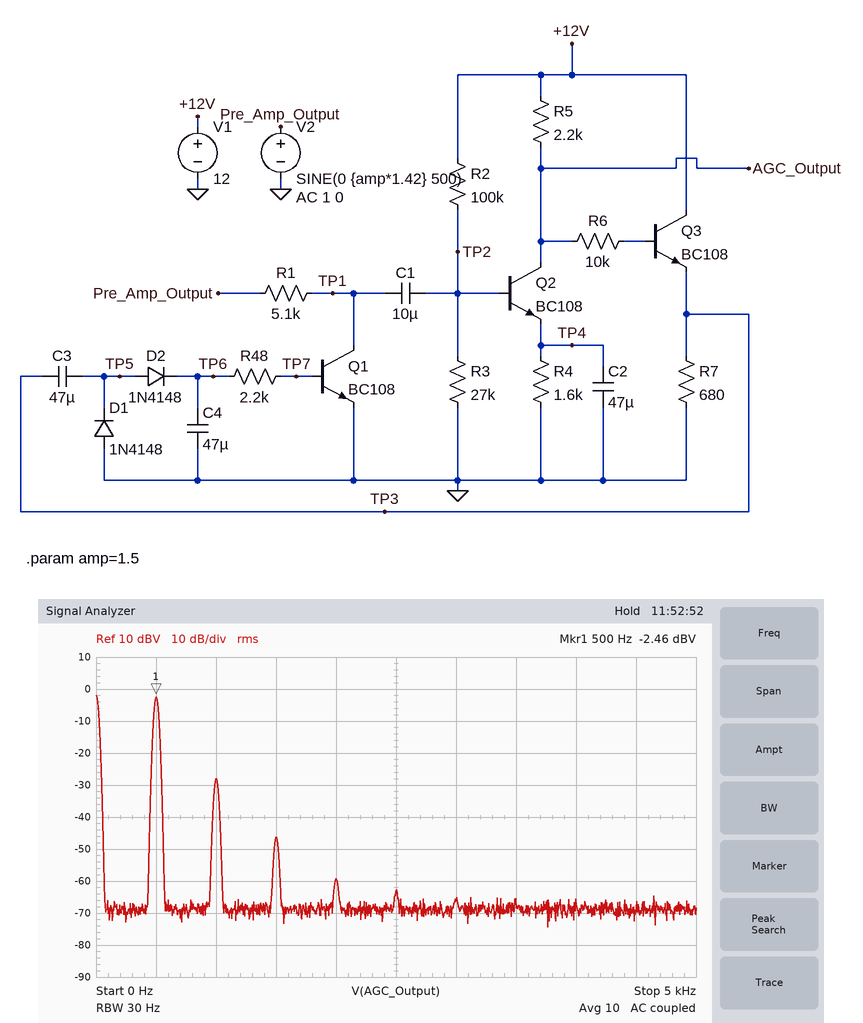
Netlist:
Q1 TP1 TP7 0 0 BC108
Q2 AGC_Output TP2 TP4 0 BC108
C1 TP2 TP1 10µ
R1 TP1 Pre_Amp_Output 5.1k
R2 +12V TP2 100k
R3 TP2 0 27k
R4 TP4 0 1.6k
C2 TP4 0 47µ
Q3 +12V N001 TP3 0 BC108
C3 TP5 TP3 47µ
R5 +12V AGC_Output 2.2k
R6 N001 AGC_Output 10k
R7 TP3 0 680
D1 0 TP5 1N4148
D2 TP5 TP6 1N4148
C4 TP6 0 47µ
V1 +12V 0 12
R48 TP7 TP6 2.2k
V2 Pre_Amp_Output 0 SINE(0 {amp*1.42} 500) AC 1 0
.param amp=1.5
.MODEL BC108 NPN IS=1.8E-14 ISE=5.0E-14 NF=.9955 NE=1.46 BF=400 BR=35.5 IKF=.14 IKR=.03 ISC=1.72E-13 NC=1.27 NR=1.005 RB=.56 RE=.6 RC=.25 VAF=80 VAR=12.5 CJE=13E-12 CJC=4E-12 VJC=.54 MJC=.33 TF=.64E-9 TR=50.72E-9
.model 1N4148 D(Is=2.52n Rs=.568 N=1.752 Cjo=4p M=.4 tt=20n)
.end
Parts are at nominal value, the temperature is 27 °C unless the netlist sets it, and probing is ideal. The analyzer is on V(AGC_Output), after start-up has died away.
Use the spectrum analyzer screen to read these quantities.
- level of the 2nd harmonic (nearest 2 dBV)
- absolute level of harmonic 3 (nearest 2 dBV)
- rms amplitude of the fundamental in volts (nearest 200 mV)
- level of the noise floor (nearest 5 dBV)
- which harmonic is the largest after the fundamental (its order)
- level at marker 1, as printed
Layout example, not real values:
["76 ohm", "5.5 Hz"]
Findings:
["-28 dBV", "-46 dBV", "800 mV", "-70 dBV", "2", "-2.46 dBV"]
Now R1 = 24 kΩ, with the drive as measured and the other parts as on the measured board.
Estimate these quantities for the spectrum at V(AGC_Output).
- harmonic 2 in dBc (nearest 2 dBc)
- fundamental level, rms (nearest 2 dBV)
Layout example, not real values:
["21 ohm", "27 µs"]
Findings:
["-24 dBc", "-4 dBV"]
